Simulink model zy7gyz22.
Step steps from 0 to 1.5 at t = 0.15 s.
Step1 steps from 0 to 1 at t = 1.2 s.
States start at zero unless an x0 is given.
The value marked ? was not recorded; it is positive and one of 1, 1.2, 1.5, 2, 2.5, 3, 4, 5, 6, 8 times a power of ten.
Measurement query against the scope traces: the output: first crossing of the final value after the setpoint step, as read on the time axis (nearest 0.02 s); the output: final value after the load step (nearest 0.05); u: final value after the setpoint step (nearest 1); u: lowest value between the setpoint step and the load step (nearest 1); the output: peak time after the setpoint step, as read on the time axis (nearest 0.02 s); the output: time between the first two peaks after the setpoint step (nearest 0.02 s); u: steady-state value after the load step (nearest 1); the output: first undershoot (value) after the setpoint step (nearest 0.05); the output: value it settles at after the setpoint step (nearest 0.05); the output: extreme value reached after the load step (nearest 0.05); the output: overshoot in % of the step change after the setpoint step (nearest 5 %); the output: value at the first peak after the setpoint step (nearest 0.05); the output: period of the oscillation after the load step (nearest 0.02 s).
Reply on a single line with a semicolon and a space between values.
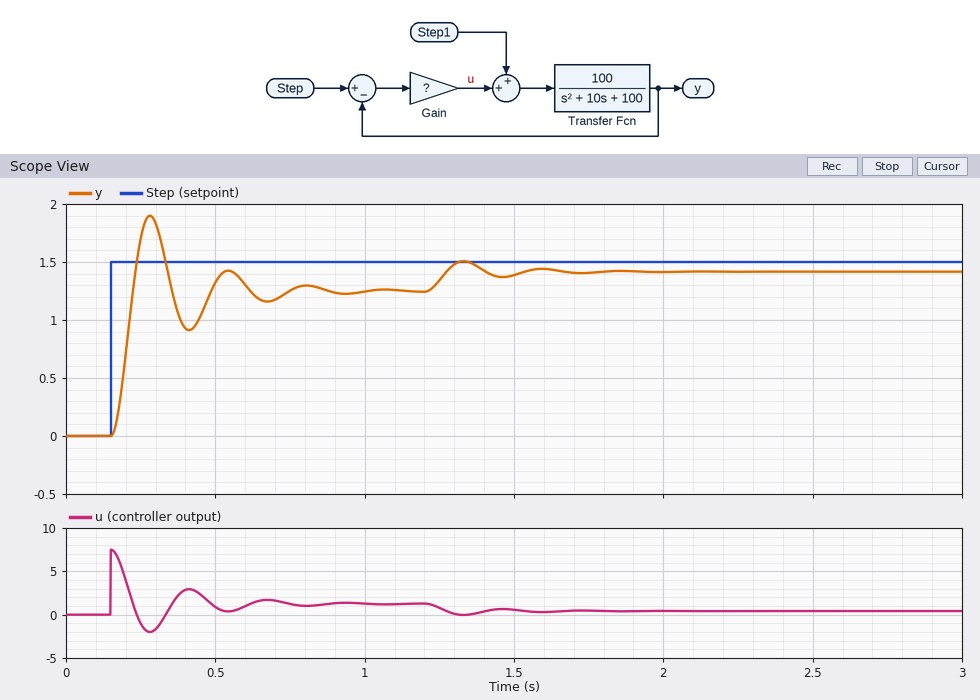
0.22 s; 1.40; 1; -2; 0.28 s; 0.26 s; 0; 0.90; 1.25; 1.50; 50 %; 1.90; 0.26 s
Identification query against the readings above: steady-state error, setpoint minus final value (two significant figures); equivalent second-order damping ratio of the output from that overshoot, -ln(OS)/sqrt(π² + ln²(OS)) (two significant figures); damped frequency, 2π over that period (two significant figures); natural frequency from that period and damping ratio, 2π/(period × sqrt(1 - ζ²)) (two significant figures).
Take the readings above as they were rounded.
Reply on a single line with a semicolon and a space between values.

0.25; 0.22; 24 rad/s; 25 rad/s
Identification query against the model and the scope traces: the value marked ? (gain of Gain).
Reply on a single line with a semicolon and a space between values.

5
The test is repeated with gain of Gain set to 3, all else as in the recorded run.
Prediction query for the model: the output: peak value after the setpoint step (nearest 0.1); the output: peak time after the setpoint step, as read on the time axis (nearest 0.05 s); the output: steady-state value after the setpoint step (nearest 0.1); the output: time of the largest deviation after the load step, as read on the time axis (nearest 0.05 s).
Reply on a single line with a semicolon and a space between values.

1.6; 0.30 s; 1.1; 1.35 s
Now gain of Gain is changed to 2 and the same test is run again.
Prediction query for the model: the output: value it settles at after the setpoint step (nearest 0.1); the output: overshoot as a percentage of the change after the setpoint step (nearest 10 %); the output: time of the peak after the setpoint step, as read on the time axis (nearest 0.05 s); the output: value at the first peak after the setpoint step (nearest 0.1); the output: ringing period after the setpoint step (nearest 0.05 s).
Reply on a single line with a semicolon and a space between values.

1.0; 40 %; 0.35 s; 1.4; 0.40 s
